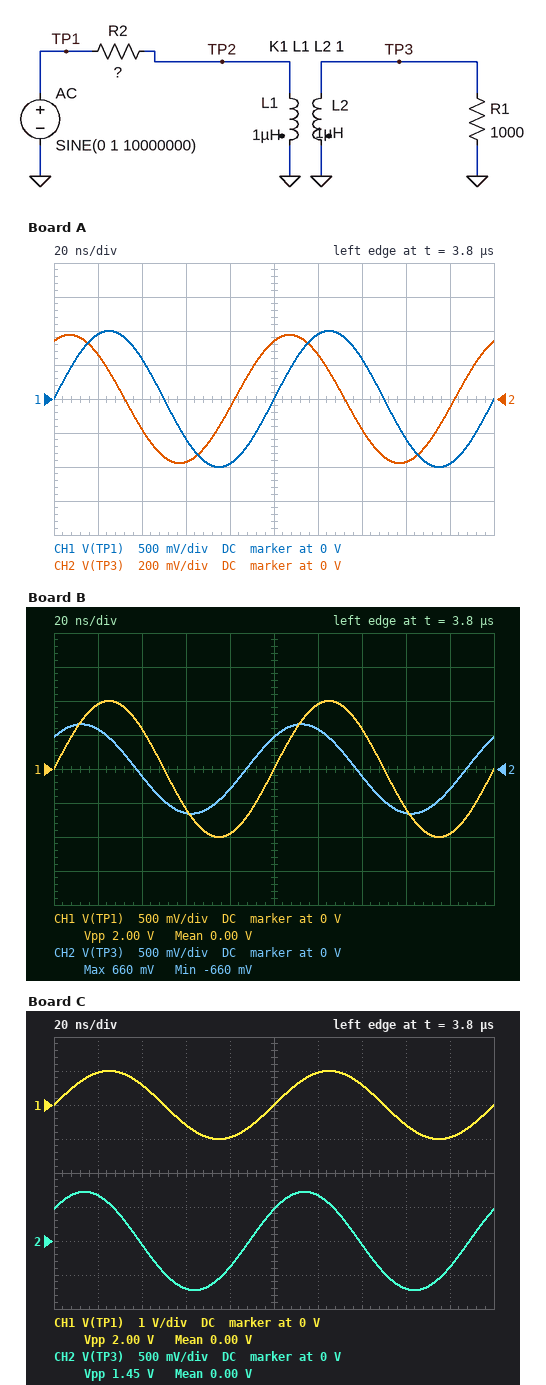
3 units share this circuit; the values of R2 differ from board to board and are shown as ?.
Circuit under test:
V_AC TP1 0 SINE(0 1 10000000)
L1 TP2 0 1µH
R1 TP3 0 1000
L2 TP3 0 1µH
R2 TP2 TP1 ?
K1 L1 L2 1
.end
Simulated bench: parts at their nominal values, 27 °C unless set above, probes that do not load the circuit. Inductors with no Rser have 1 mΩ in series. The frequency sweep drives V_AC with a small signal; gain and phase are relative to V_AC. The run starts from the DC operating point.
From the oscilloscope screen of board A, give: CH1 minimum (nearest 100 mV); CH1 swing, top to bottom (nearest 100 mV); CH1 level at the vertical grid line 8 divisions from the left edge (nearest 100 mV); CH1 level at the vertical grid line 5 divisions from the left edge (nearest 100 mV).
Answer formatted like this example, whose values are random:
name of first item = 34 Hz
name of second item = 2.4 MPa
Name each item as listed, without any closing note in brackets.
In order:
CH1 minimum = -1.0 V
CH1 swing, top to bottom = 2.0 V
CH1 level at the vertical grid line 8 divisions from the left edge = -600 mV
CH1 level at the vertical grid line 5 divisions from the left edge = 0 V
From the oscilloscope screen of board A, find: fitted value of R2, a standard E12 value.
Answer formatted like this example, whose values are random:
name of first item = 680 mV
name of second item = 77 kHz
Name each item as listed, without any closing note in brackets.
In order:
fitted value of R2, a standard E12 value = 150 Ω
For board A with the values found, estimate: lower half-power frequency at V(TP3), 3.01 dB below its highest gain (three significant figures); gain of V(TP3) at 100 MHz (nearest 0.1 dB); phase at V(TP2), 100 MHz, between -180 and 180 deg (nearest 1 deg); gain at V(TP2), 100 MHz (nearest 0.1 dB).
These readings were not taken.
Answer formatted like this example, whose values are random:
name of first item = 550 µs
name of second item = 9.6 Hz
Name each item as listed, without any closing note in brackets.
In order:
lower half-power frequency at V(TP3), 3.01 dB below its highest gain = 20.8 MHz
gain of V(TP3) at 100 MHz = -1.4 dB
phase at V(TP2), 100 MHz, between -180 and 180 deg = 12 deg
gain at V(TP2), 100 MHz = -1.4 dB
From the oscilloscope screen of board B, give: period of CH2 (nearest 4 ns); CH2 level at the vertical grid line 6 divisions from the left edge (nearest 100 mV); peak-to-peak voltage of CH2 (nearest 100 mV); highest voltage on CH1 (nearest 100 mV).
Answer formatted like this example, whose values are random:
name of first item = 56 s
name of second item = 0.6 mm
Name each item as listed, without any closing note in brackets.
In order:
period of CH2 = 100 ns
CH2 level at the vertical grid line 6 divisions from the left edge = 600 mV
peak-to-peak voltage of CH2 = 1.3 V
highest voltage on CH1 = 1.0 V
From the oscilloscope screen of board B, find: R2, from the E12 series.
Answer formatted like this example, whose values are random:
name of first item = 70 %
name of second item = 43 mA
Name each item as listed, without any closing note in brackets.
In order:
R2, from the E12 series = 68 Ω
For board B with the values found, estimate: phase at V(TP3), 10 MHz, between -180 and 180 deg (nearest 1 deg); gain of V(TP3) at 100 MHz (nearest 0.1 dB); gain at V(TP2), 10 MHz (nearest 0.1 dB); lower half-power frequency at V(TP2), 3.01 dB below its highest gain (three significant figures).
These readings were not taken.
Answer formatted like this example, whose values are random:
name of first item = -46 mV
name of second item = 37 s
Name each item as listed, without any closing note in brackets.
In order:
phase at V(TP3), 10 MHz, between -180 and 180 deg = 45 deg
gain of V(TP3) at 100 MHz = -0.6 dB
gain at V(TP2), 10 MHz = -3.6 dB
lower half-power frequency at V(TP2), 3.01 dB below its highest gain = 10.1 MHz
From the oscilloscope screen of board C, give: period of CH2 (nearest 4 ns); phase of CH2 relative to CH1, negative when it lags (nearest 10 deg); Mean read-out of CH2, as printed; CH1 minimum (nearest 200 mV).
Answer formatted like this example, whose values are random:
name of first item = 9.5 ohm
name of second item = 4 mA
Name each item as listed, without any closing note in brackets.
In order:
period of CH2 = 100 ns
phase of CH2 relative to CH1, negative when it lags = 40 deg
Mean read-out of CH2, as printed = 0.00 V
CH1 minimum = -1.0 V
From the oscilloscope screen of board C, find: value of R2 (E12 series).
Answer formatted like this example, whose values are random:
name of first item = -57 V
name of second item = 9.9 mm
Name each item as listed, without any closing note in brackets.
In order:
value of R2 = 56 Ω
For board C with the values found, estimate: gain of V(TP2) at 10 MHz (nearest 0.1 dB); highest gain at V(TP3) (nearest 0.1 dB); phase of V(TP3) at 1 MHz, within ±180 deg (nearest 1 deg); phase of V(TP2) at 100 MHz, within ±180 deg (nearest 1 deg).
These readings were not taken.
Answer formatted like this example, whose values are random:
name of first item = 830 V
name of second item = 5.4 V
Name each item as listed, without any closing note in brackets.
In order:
gain of V(TP2) at 10 MHz = -2.8 dB
highest gain at V(TP3) = -0.5 dB
phase of V(TP3) at 1 MHz, within ±180 deg = 83 deg
phase of V(TP2) at 100 MHz, within ±180 deg = 5 deg
